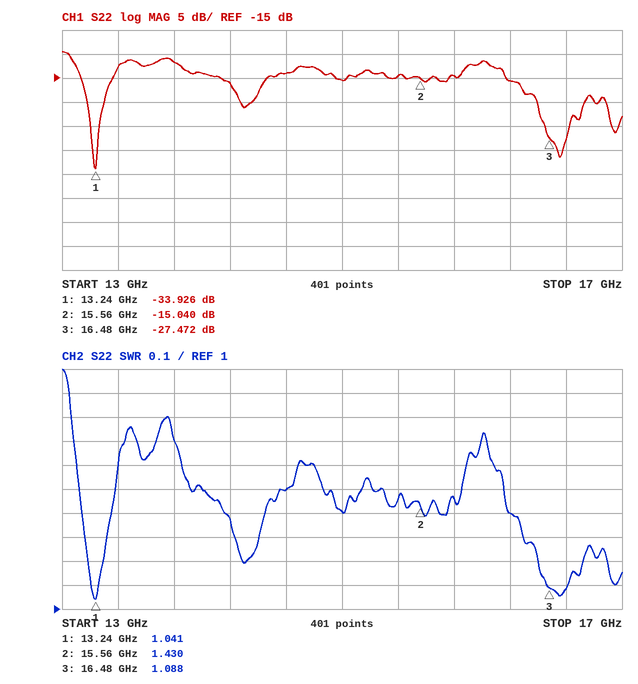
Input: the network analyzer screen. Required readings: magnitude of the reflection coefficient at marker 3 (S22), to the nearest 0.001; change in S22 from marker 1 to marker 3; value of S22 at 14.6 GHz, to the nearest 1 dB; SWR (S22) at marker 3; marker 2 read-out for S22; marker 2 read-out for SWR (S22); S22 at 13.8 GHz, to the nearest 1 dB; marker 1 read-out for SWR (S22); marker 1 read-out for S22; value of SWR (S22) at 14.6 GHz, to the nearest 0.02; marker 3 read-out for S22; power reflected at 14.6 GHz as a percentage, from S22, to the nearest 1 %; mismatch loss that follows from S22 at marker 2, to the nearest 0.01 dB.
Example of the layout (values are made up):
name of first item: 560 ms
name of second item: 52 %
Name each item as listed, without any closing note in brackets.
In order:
magnitude of the reflection coefficient at marker 3 (S22), to the nearest 0.001: 0.042
change in S22 from marker 1 to marker 3: 6.454 dB
value of S22 at 14.6 GHz, to the nearest 1 dB: -14 dB
SWR (S22) at marker 3: 1.088
marker 2 read-out for S22: -15.040 dB
marker 2 read-out for SWR: 1.430
S22 at 13.8 GHz, to the nearest 1 dB: -12 dB
marker 1 read-out for SWR: 1.041
marker 1 read-out for S22: -33.926 dB
value of SWR (S22) at 14.6 GHz, to the nearest 0.02: 1.50
marker 3 read-out for S22: -27.472 dB
power reflected at 14.6 GHz as a percentage, from S22, to the nearest 1 %: 4 %
mismatch loss that follows from S22 at marker 2, to the nearest 0.01 dB: 0.14 dB
